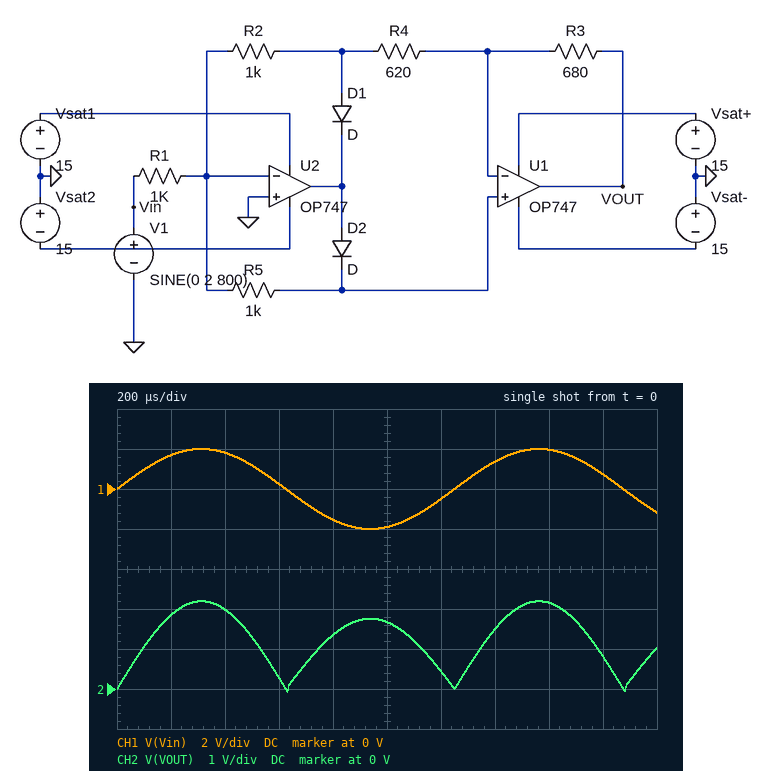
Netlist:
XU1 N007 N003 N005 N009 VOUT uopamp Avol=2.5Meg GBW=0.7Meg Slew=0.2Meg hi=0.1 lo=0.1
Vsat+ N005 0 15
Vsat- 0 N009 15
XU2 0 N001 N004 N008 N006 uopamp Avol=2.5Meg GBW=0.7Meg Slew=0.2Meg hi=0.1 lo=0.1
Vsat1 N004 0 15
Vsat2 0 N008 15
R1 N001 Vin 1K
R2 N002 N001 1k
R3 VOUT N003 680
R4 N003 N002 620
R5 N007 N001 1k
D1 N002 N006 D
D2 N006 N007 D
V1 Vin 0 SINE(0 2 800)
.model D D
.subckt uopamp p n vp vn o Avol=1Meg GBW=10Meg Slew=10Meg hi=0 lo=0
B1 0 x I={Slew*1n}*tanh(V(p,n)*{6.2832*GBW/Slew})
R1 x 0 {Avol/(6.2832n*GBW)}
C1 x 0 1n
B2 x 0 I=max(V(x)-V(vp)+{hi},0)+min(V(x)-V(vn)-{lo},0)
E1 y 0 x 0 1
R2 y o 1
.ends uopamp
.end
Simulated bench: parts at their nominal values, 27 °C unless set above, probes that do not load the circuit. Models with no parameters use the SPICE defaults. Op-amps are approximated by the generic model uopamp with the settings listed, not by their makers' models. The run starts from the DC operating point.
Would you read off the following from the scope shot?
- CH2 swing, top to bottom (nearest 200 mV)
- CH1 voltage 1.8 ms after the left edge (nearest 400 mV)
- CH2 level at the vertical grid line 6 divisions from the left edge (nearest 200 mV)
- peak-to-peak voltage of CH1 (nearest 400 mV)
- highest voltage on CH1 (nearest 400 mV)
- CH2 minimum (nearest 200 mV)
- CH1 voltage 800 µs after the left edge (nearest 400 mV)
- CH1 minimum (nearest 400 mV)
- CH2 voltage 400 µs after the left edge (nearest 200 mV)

2.2 V
800 mV
400 mV
4.0 V
2.0 V
0 V
-1.6 V
-2.0 V
2.0 V
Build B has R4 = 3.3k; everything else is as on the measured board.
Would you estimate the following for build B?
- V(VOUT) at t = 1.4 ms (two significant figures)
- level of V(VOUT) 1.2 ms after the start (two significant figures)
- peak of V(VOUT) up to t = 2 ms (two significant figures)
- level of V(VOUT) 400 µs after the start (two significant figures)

280 mV
470 mV
1.9 V
370 mV
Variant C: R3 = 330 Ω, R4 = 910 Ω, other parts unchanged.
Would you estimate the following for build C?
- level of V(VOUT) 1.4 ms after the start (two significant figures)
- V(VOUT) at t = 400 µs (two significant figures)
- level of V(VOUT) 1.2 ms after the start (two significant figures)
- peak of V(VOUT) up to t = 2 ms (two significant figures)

500 mV
660 mV
390 mV
1.5 V
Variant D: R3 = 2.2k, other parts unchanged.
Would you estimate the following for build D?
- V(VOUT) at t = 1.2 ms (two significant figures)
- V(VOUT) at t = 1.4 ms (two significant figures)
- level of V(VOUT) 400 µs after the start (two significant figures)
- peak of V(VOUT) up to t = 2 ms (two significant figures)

730 mV
4.8 V
6.4 V
7.1 V
